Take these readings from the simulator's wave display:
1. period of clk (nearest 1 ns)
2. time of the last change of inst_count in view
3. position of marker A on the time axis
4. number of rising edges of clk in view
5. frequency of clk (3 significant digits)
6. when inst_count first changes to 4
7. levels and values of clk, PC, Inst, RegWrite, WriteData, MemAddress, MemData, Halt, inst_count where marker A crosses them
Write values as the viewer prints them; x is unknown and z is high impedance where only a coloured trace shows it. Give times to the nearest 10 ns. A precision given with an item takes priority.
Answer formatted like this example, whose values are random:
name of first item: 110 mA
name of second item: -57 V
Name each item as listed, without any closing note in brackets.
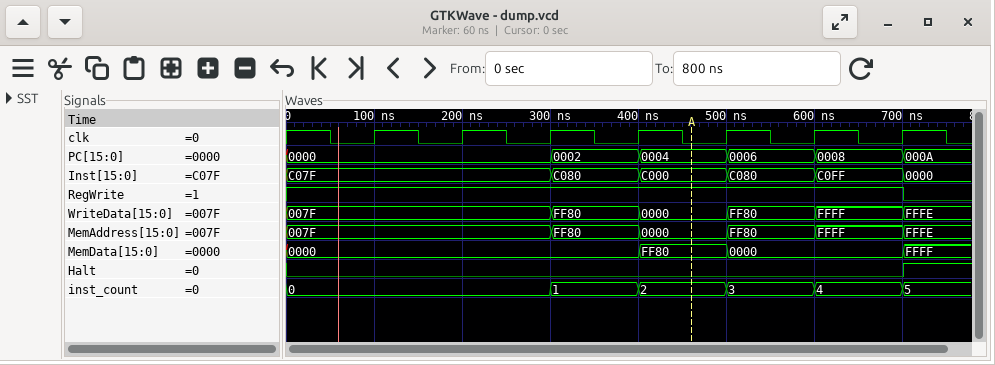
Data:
period of clk: 100 ns
time of the last change of inst_count in view: 700 ns
position of marker A on the time axis: 460 ns
number of rising edges of clk in view: 7
frequency of clk: 10.0 MHz
when inst_count first changes to 4: 600 ns
levels and values of clk, PC, Inst, RegWrite, WriteData, MemAddress, MemData, Halt, inst_count where marker A crosses them: clk=0, PC=0004, Inst=C000, RegWrite=1, WriteData=0000, MemAddress=0000, MemData=FF80, Halt=0, inst_count=2
